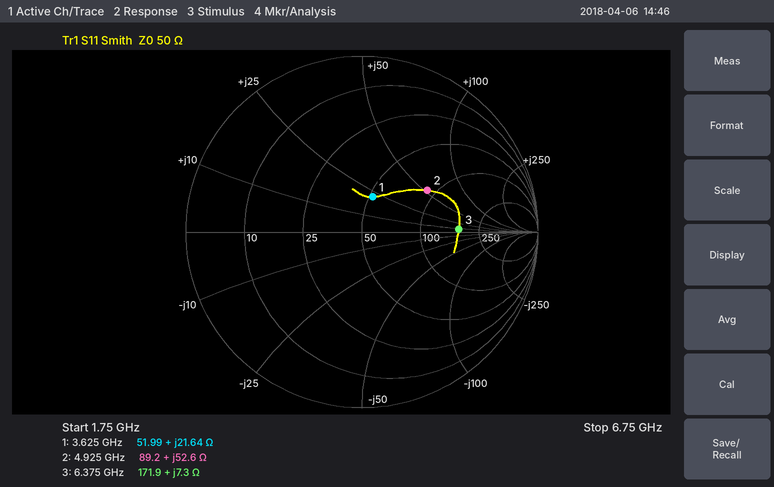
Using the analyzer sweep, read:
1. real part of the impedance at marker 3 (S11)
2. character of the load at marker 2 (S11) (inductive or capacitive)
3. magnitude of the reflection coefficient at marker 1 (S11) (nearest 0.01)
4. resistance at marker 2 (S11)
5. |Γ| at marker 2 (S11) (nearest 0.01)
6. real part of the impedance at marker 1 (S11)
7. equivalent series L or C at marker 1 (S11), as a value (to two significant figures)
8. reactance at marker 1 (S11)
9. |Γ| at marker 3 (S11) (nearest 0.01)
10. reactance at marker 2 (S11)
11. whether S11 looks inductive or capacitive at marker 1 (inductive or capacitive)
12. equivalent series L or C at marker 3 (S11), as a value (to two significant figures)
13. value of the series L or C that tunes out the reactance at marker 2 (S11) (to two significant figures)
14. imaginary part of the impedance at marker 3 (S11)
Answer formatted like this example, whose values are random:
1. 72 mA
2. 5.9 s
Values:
1. 171.9 Ω
2. inductive
3. 0.21
4. 89.2 Ω
5. 0.44
6. 51.99 Ω
7. 950 pH
8. +21.64 Ω
9. 0.55
10. +52.6 Ω
11. inductive
12. 180 pH
13. 610 fF
14. +7.3 Ω
